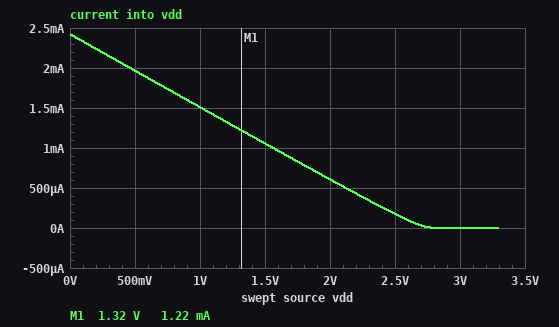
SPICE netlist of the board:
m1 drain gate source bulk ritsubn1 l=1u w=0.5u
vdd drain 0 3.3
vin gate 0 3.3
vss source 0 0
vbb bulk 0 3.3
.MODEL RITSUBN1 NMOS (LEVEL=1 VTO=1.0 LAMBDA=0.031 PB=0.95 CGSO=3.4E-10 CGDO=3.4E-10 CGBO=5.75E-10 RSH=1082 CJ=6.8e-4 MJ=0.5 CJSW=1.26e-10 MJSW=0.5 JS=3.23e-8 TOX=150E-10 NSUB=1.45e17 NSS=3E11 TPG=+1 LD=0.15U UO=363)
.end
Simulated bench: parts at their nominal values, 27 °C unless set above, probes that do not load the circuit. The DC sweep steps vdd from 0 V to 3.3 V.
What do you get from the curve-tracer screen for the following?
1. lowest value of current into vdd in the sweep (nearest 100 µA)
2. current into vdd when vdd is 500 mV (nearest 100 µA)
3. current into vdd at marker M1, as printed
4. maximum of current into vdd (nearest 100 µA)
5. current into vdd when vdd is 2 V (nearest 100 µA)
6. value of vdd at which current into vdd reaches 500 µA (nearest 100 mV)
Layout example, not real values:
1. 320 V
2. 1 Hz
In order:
1. 0 A
2. 2.0 mA
3. 1.22 mA
4. 2.4 mA
5. 600 µA
6. 2.1 V
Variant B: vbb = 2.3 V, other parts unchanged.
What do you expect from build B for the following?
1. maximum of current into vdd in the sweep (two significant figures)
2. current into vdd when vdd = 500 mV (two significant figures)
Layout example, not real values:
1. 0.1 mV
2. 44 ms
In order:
1. 1.5 mA
2. 1.1 mA
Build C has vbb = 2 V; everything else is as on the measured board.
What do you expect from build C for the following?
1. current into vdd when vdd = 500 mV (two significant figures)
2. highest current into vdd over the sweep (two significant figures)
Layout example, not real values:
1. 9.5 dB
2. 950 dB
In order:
1. 790 µA
2. 1.2 mA
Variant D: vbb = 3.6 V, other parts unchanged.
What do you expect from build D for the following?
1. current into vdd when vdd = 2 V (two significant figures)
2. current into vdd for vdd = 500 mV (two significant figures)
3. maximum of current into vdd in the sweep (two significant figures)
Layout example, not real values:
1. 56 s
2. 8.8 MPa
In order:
1. 880 µA
2. 2.2 mA
3. 2.7 mA
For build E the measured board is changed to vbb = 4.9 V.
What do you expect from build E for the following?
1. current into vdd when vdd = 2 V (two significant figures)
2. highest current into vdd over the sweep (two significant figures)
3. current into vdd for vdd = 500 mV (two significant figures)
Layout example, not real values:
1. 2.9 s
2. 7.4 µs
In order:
1. 2.1 mA
2. 3.9 mA
3. 3.4 mA
